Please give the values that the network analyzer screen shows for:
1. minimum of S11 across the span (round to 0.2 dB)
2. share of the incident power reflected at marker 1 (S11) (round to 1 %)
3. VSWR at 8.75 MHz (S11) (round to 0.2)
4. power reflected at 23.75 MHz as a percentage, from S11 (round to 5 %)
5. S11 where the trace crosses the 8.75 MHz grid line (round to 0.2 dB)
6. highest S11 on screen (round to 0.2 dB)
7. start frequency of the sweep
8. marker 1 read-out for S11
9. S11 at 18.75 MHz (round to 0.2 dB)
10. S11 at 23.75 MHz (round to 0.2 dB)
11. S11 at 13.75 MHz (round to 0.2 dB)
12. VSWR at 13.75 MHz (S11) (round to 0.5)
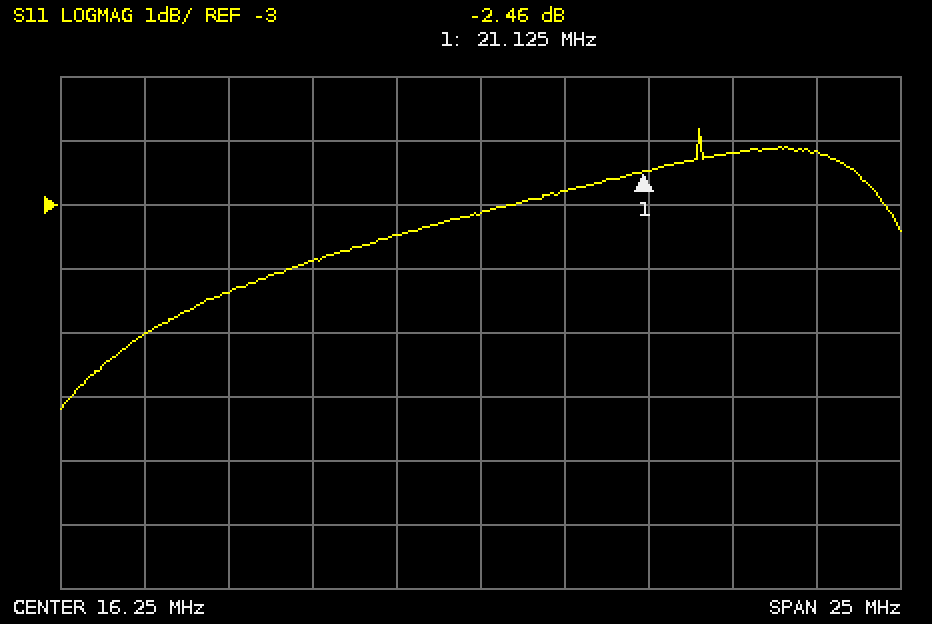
-6.2 dB
57 %
4.0
60 %
-4.4 dB
-1.8 dB
3.75 MHz
-2.46 dB
-2.8 dB
-2.2 dB
-3.4 dB
5.0
